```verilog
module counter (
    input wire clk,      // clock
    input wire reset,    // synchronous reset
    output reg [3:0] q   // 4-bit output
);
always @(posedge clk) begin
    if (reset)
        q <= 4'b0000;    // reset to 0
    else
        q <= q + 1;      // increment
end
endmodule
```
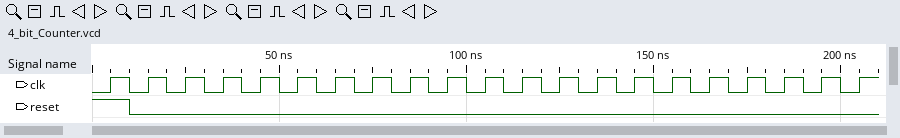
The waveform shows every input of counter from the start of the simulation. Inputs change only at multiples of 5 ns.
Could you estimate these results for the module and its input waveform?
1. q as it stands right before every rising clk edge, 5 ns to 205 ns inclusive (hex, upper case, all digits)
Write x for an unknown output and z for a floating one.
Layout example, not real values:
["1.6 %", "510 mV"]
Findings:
["x, 0, 1, 2, 3, 4, 5, 6, 7, 8, 9, A, B, C, D, E, F, 0, 1, 2, 3"]
